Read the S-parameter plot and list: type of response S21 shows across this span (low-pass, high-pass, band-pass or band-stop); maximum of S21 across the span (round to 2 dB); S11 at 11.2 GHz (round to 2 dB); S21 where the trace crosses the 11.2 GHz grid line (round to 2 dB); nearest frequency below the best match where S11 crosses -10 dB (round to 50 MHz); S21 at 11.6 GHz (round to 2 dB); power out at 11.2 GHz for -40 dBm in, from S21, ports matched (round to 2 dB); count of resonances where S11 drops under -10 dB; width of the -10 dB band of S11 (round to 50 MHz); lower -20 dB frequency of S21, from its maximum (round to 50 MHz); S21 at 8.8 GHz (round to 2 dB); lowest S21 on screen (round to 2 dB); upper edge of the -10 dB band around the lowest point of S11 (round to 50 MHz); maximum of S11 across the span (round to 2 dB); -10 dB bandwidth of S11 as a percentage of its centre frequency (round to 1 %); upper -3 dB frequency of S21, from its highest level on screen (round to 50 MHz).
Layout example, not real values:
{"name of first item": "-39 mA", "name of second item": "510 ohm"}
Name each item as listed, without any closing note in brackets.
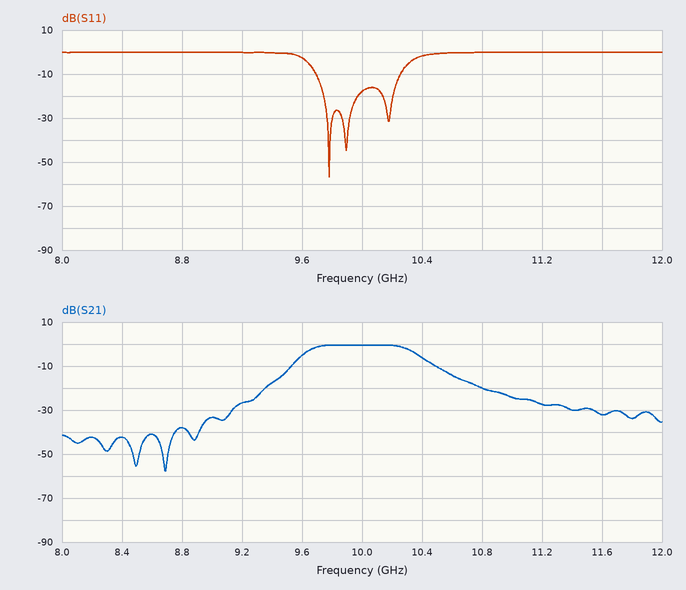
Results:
{"type of response S21 shows across this span": "band-pass", "maximum of S21 across the span": "0 dB", "S11 at 11.2 GHz": "0 dB", "S21 where the trace crosses the 11.2 GHz grid line": "-28 dB", "nearest frequency below the best match where S11 crosses -10 dB": "9.70 GHz", "S21 at 11.6 GHz": "-32 dB", "power out at 11.2 GHz for -40 dBm in, from S21, ports matched": "-68 dBm", "count of resonances where S11 drops under -10 dB": "3", "width of the -10 dB band of S11": "550 MHz", "lower -20 dB frequency of S21, from its maximum": "9.35 GHz", "S21 at 8.8 GHz": "-38 dB", "lowest S21 on screen": "-58 dB", "upper edge of the -10 dB band around the lowest point of S11": "10.25 GHz", "maximum of S11 across the span": "0 dB", "-10 dB bandwidth of S11 as a percentage of its centre frequency": "6 %", "upper -3 dB frequency of S21, from its highest level on screen": "10.35 GHz"}
